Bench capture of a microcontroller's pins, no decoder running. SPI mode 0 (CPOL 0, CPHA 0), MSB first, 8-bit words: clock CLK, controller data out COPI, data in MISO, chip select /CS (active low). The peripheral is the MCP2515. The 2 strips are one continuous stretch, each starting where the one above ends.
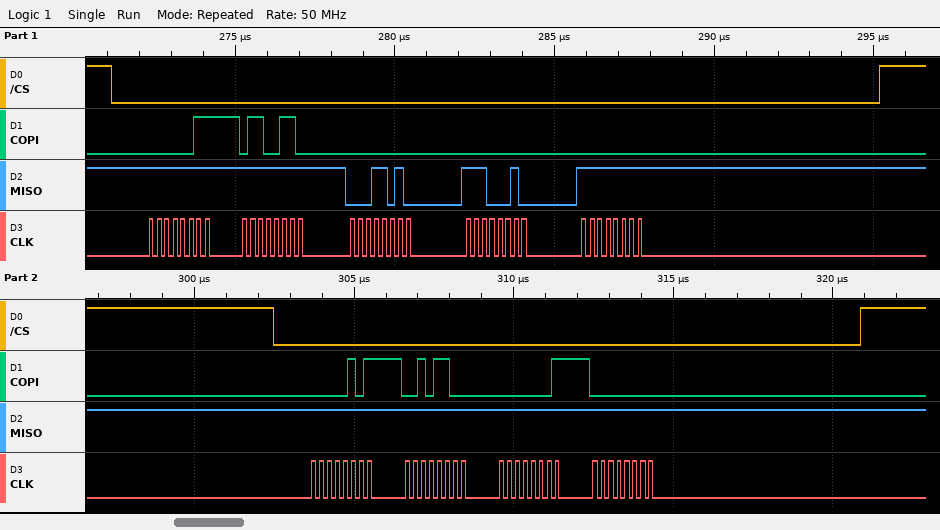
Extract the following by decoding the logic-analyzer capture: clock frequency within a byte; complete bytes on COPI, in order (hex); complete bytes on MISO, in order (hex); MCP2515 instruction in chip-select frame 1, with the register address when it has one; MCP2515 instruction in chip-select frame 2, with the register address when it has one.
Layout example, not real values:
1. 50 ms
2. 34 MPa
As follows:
1. 4 MHz
2. 03 66 00 00 00 05 2C 01 00
3. FF FF 1A E2 FF FF FF FF FF
4. READ 0x66
5. BIT MODIFY 0x2C
